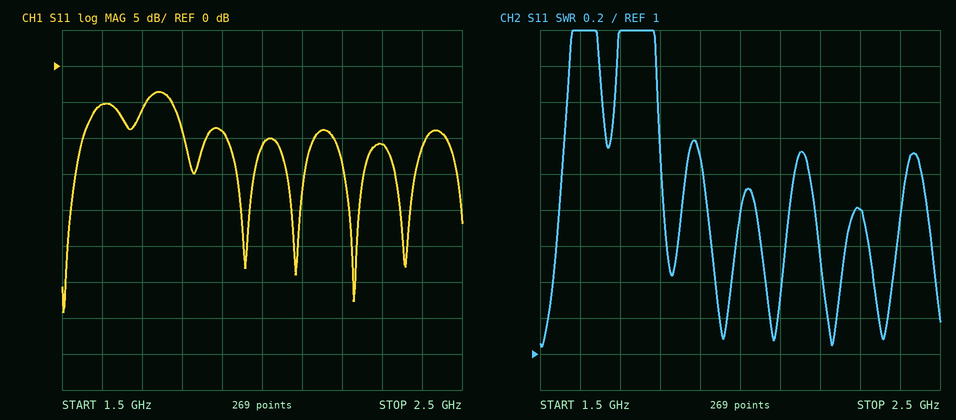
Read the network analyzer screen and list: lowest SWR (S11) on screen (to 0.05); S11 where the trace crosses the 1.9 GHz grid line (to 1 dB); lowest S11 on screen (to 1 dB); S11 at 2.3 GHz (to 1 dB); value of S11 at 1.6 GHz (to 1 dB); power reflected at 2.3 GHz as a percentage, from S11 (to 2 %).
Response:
1.05
-9 dB
-34 dB
-11 dB
-5 dB
8 %
